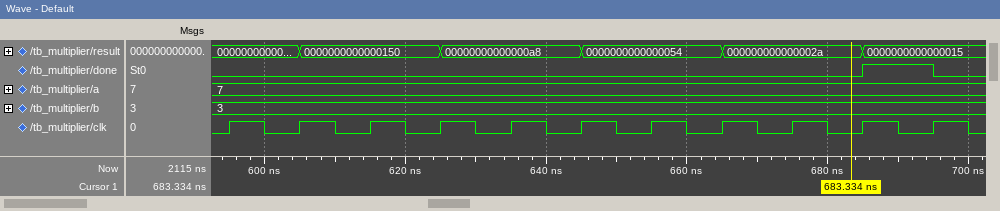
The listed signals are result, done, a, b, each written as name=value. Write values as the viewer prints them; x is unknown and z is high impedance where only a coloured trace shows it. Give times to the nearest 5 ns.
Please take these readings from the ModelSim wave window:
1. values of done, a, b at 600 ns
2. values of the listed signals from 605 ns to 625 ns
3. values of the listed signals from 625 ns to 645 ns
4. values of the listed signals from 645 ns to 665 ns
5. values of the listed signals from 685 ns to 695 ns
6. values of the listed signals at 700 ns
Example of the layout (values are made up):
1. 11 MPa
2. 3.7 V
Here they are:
1. done=0, a=7, b=3
2. result=0000000000000150, done=0, a=7, b=3
3. result=00000000000000a8, done=0, a=7, b=3
4. result=0000000000000054, done=0, a=7, b=3
5. result=0000000000000015, done=1, a=7, b=3
6. result=0000000000000015, done=0, a=7, b=3
